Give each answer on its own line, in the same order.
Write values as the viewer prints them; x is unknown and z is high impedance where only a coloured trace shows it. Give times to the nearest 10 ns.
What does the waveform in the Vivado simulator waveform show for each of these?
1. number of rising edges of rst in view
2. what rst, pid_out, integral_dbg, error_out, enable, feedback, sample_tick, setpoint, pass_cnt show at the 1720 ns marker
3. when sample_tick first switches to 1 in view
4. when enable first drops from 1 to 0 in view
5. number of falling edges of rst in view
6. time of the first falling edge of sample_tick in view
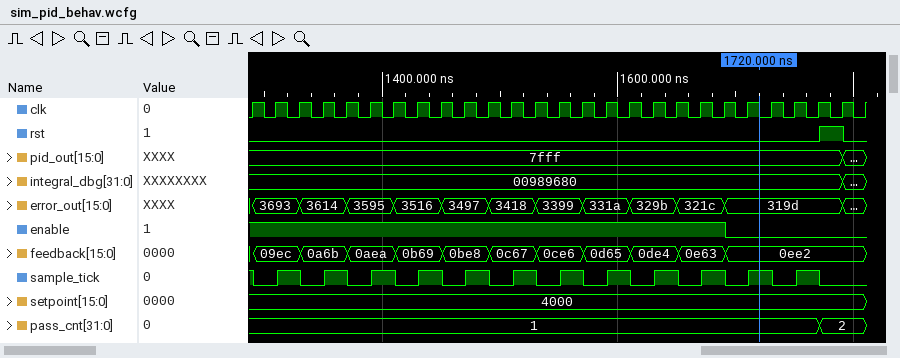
1
rst=0, pid_out=7fff, integral_dbg=00989680, error_out=319d, enable=0, feedback=0ee2, sample_tick=1, setpoint=4000, pass_cnt=1
1310 ns
1690 ns
1
1290 ns
